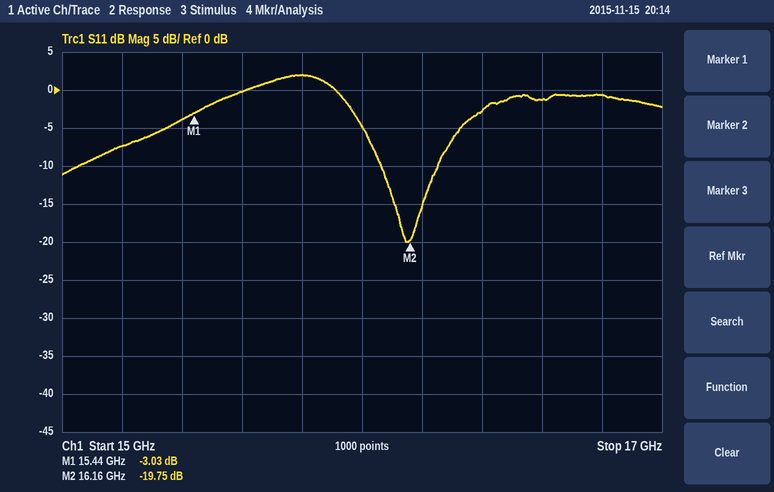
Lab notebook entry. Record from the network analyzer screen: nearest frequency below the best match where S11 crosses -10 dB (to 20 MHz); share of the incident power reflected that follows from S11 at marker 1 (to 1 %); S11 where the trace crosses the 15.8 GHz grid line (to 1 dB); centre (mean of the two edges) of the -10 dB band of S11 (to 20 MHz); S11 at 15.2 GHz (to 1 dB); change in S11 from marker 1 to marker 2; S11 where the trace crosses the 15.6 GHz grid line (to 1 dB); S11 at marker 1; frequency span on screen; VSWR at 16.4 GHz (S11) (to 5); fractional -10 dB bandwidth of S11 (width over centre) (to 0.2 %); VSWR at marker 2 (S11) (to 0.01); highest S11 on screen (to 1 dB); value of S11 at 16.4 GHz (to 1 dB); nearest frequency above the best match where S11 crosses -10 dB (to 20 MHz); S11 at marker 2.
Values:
16.06 GHz
50 %
2 dB
16.16 GHz
-7 dB
-16.72 dB
0 dB
-3.03 dB
2 GHz
5
1.2 %
1.23
2 dB
-3 dB
16.26 GHz
-19.75 dB
